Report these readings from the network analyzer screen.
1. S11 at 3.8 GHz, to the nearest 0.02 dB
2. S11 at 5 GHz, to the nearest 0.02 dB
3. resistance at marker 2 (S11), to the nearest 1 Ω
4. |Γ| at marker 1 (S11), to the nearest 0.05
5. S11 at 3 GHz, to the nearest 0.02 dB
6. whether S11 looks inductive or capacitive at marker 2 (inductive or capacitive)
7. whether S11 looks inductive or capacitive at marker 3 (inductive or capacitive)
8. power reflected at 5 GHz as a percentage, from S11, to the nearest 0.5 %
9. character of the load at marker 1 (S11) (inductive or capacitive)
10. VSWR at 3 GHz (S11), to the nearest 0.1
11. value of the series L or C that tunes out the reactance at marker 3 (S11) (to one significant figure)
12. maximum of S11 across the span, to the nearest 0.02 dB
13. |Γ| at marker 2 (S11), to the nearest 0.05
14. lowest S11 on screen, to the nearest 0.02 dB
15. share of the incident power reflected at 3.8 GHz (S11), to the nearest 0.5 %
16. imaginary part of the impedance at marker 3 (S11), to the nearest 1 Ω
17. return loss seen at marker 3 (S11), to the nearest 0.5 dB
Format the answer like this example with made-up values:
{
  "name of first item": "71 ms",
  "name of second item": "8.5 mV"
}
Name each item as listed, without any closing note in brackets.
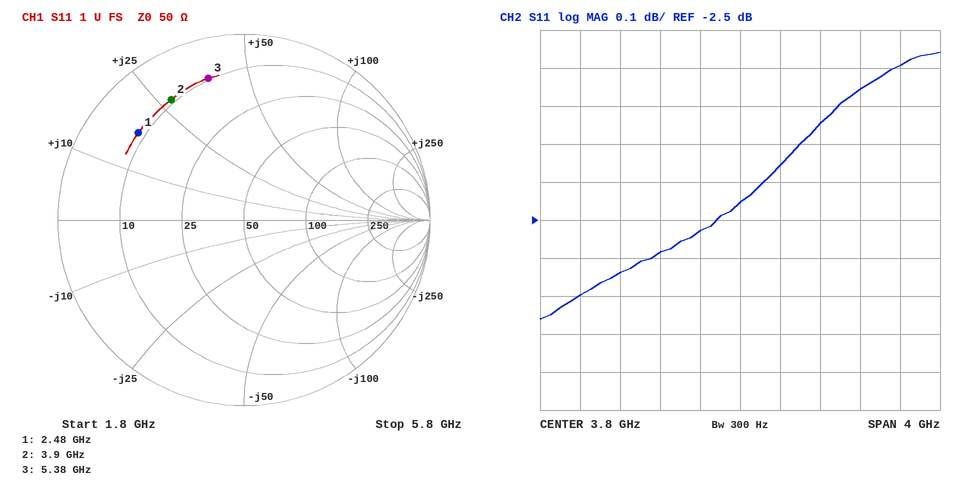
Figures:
{
  "S11 at 3.8 GHz, to the nearest 0.02 dB": "-2.46 dB",
  "S11 at 5 GHz, to the nearest 0.02 dB": "-2.16 dB",
  "resistance at marker 2 (S11), to the nearest 1 Ω": "9 Ω",
  "|Γ| at marker 1 (S11), to the nearest 0.05": "0.75",
  "S11 at 3 GHz, to the nearest 0.02 dB": "-2.58 dB",
  "whether S11 looks inductive or capacitive at marker 2": "inductive",
  "whether S11 looks inductive or capacitive at marker 3": "inductive",
  "power reflected at 5 GHz as a percentage, from S11, to the nearest 0.5 %": "61.0 %",
  "character of the load at marker 1 (S11)": "inductive",
  "VSWR at 3 GHz (S11), to the nearest 0.1": "6.8",
  "value of the series L or C that tunes out the reactance at marker 3 (S11)": "800 fF",
  "maximum of S11 across the span, to the nearest 0.02 dB": "-2.06 dB",
  "|Γ| at marker 2 (S11), to the nearest 0.05": "0.75",
  "lowest S11 on screen, to the nearest 0.02 dB": "-2.76 dB",
  "share of the incident power reflected at 3.8 GHz (S11), to the nearest 0.5 %": "57.0 %",
  "imaginary part of the impedance at marker 3 (S11), to the nearest 1 Ω": "+38 Ω",
  "return loss seen at marker 3 (S11), to the nearest 0.5 dB": "2.0 dB"
}
